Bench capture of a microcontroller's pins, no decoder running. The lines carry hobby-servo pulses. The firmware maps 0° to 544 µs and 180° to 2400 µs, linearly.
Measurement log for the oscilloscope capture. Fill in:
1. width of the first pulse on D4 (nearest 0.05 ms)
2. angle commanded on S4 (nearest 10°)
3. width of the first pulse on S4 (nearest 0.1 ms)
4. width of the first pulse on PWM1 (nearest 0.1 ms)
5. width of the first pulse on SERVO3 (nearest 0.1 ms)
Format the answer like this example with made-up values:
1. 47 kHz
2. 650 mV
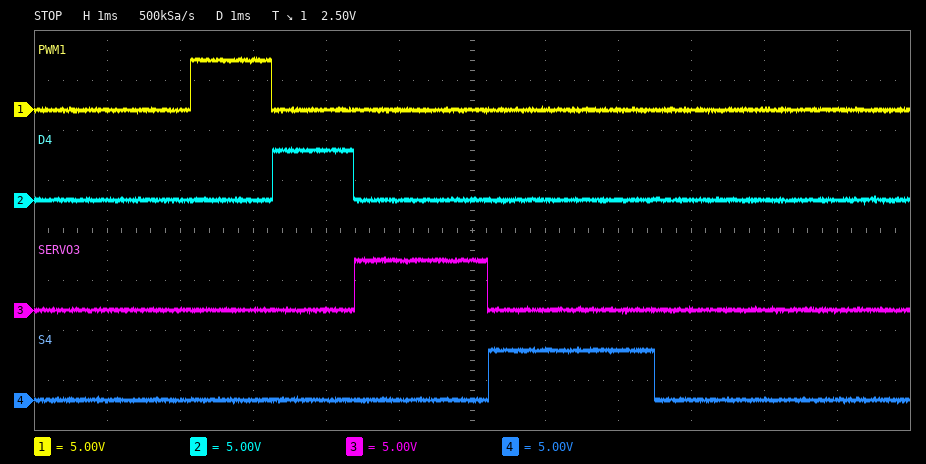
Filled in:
1. 1.10 ms
2. 170°
3. 2.3 ms
4. 1.1 ms
5. 1.8 ms
